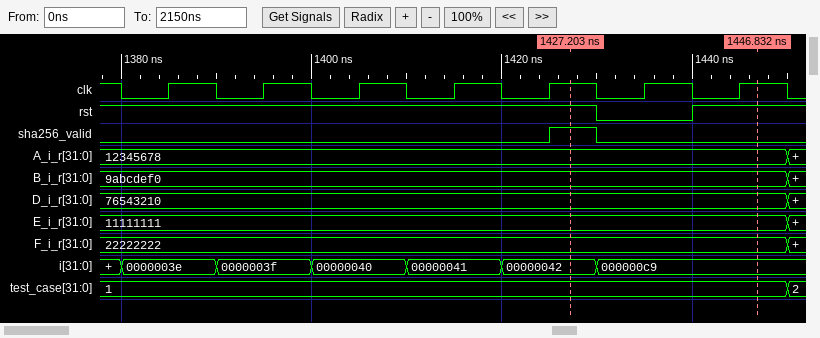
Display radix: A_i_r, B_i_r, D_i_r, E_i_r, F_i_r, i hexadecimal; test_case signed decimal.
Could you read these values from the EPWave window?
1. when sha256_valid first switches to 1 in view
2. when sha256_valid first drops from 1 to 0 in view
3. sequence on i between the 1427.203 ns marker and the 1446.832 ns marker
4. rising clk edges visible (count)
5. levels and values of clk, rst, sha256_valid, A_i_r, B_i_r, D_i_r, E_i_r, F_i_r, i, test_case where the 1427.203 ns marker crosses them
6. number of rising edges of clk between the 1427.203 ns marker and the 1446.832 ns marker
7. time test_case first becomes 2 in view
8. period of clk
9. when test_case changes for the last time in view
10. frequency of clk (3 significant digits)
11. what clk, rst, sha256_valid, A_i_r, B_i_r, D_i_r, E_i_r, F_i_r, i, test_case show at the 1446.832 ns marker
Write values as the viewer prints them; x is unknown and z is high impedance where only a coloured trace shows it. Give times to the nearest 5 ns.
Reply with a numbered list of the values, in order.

1. 1425 ns
2. 1430 ns
3. 00000042, 000000c9
4. 7
5. clk=1, rst=1, sha256_valid=1, A_i_r=12345678, B_i_r=9abcdef0, D_i_r=76543210, E_i_r=11111111, F_i_r=22222222, i=00000042, test_case=1
6. 2
7. 1450 ns
8. 10 ns
9. 1450 ns
10. 100 MHz
11. clk=1, rst=1, sha256_valid=0, A_i_r=12345678, B_i_r=9abcdef0, D_i_r=76543210, E_i_r=11111111, F_i_r=22222222, i=000000c9, test_case=1
